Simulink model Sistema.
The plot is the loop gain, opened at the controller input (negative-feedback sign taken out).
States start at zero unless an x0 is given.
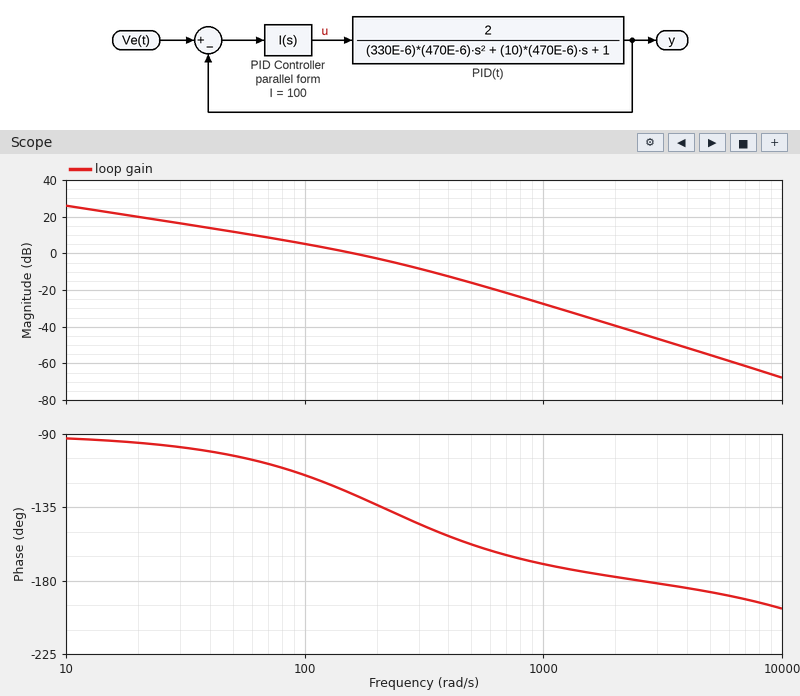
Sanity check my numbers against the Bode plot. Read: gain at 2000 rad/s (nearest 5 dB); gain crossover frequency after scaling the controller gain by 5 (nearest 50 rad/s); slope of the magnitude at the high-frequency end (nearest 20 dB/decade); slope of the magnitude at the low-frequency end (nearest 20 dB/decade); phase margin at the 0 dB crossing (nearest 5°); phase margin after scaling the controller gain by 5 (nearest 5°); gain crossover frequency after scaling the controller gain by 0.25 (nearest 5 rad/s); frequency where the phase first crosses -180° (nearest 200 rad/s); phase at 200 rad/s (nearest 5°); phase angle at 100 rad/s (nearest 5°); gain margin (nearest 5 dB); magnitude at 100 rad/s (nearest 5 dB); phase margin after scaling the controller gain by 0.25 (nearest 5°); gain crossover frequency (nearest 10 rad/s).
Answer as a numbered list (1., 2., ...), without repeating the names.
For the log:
1. -40 dB
2. 450 rad/s
3. -40 dB/decade
4. -20 dB/decade
5. 55°
6. 25°
7. 50 rad/s
8. 2600 rad/s
9. -135°
10. -115°
11. 45 dB
12. 5 dB
13. 75°
14. 160 rad/s
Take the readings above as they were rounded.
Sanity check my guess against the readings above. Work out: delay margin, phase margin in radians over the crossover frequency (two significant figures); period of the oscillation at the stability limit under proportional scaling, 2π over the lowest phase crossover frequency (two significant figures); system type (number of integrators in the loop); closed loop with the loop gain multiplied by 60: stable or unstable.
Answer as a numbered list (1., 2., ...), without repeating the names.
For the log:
1. 0.0060 s
2. 0.0024 s
3. 1
4. stable
